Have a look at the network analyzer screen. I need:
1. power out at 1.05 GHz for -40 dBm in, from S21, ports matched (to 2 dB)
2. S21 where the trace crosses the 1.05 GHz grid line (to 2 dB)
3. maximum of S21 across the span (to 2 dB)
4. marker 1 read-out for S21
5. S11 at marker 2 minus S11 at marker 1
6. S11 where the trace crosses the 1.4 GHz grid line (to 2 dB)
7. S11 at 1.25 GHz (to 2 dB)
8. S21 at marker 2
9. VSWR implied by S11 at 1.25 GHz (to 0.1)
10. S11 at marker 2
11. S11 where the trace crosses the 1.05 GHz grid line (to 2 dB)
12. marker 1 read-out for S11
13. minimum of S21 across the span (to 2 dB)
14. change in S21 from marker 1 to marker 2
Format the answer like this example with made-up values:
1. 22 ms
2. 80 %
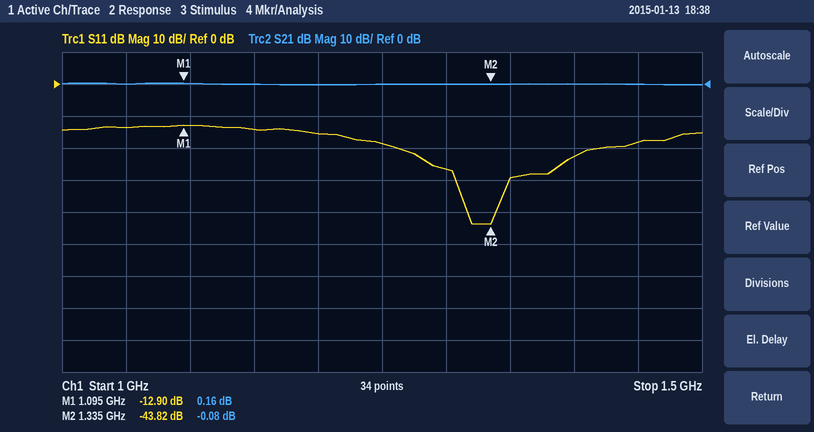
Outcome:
1. -40 dBm
2. 0 dB
3. 0 dB
4. 0.16 dB
5. -30.92 dB
6. -22 dB
7. -18 dB
8. -0.08 dB
9. 1.3
10. -43.82 dB
11. -14 dB
12. -12.90 dB
13. 0 dB
14. -0.24 dB
